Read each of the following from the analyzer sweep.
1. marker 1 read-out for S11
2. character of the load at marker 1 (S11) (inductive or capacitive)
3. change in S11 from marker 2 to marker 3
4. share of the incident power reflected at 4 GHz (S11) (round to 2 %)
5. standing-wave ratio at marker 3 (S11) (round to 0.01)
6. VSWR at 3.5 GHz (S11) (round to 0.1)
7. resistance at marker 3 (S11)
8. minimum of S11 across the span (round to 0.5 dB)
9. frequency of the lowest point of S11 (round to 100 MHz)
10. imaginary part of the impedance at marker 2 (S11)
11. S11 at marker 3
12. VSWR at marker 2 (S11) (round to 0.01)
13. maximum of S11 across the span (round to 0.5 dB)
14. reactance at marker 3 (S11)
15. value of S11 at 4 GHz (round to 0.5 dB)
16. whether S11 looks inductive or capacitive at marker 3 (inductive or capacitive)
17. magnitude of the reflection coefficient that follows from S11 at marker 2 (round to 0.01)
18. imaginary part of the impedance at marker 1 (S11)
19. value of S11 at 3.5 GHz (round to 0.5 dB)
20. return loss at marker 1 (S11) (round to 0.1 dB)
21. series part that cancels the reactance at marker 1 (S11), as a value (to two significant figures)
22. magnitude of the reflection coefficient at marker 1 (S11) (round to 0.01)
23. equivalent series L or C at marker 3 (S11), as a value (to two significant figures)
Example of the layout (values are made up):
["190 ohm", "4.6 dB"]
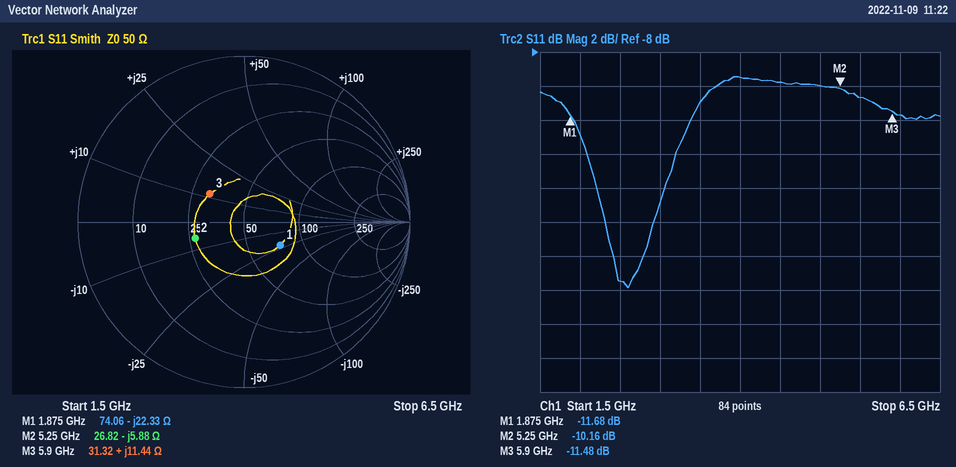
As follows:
["-11.68 dB", "capacitive", "-1.32 dB", "12 %", "1.73", "1.8", "31.32 Ω", "-22.0 dB", "2.6 GHz", "-5.88 Ω", "-11.48 dB", "1.90", "-9.5 dB", "+11.44 Ω", "-9.5 dB", "inductive", "0.31", "-22.33 Ω", "-11.0 dB", "11.7 dB", "1.9 nH", "0.26", "310 pH"]
